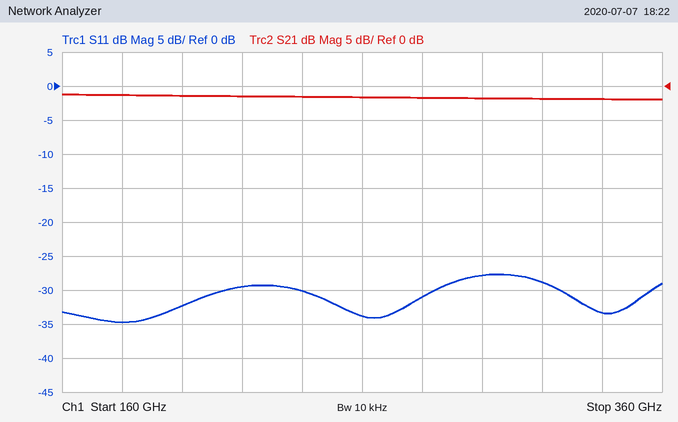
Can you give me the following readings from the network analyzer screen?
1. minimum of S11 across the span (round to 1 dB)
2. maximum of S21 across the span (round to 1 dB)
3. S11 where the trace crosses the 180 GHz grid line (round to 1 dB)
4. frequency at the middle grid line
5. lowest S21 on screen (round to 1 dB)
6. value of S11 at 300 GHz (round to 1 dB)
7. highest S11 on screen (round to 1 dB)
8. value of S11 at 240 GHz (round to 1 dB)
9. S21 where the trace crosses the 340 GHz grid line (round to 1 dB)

-35 dB
-1 dB
-35 dB
260 GHz
-2 dB
-28 dB
-28 dB
-30 dB
-2 dB
